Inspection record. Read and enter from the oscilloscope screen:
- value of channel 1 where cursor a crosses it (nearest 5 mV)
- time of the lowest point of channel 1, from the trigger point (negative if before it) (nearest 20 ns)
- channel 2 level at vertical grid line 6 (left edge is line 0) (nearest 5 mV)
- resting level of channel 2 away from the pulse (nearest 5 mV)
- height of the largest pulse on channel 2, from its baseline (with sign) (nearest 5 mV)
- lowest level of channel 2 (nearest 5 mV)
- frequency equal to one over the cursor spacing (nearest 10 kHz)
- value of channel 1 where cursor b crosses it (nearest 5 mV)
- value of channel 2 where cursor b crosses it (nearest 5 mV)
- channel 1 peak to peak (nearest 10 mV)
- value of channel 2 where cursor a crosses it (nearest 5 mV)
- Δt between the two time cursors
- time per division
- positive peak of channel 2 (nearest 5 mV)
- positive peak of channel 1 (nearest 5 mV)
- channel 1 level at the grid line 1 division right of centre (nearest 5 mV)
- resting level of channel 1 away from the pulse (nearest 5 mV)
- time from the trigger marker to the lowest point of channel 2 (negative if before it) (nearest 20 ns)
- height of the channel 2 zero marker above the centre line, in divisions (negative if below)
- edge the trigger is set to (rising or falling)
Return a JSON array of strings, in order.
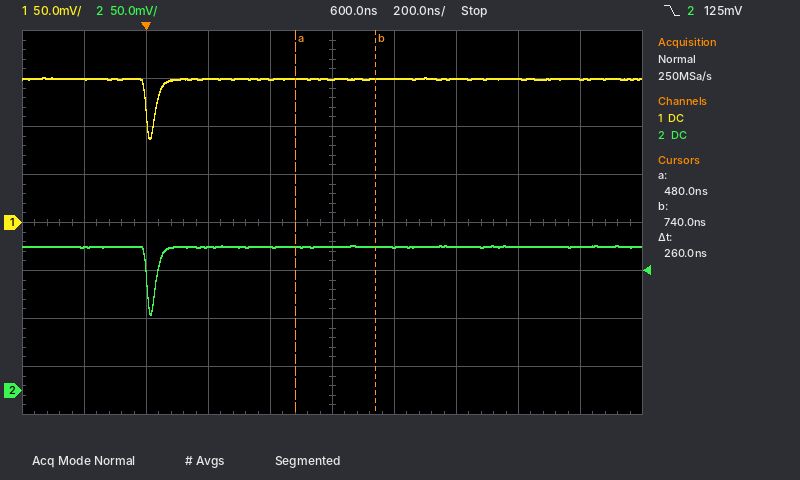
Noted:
["150 mV", "+20 ns", "150 mV", "150 mV", "-70 mV", "80 mV", "3.85 MHz", "150 mV", "150 mV", "60 mV", "150 mV", "260 ns", "200 ns", "150 mV", "150 mV", "150 mV", "150 mV", "+20 ns", "-3.5 div", "falling"]
